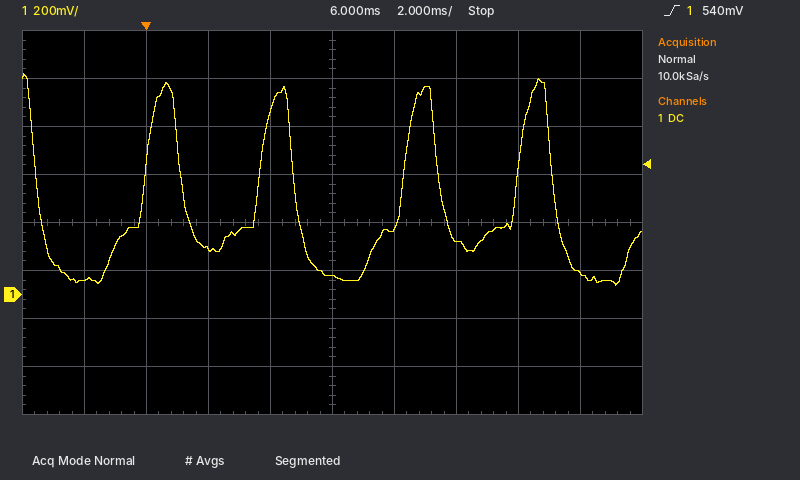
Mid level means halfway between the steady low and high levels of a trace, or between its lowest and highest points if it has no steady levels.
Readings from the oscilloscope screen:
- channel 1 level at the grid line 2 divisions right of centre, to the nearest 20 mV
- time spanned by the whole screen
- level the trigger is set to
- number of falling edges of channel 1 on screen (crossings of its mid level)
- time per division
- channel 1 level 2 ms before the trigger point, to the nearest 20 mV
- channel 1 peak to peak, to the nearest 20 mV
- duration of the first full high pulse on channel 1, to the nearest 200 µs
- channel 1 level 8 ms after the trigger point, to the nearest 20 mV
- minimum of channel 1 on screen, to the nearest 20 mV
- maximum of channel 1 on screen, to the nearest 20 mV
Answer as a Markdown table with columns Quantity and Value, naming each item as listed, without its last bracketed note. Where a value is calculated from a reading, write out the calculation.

| Quantity | Value |
|---|---|
| channel 1 level at the grid line 2 divisions right of centre, to the nearest 20 mV | 220 mV |
| time spanned by the whole screen | 20 ms |
| level the trigger is set to | 540 mV |
| number of falling edges of channel 1 on screen | 5 |
| time per division | 2 ms |
| channel 1 level 2 ms before the trigger point, to the nearest 20 mV | 60 mV |
| channel 1 peak to peak, to the nearest 20 mV | 920 mV − (40 mV) = 880 mV |
| duration of the first full high pulse on channel 1, to the nearest 200 µs | 1.2 ms |
| channel 1 level 8 ms after the trigger point, to the nearest 20 mV | 280 mV |
| minimum of channel 1 on screen, to the nearest 20 mV | 40 mV |
| maximum of channel 1 on screen, to the nearest 20 mV | 920 mV |
